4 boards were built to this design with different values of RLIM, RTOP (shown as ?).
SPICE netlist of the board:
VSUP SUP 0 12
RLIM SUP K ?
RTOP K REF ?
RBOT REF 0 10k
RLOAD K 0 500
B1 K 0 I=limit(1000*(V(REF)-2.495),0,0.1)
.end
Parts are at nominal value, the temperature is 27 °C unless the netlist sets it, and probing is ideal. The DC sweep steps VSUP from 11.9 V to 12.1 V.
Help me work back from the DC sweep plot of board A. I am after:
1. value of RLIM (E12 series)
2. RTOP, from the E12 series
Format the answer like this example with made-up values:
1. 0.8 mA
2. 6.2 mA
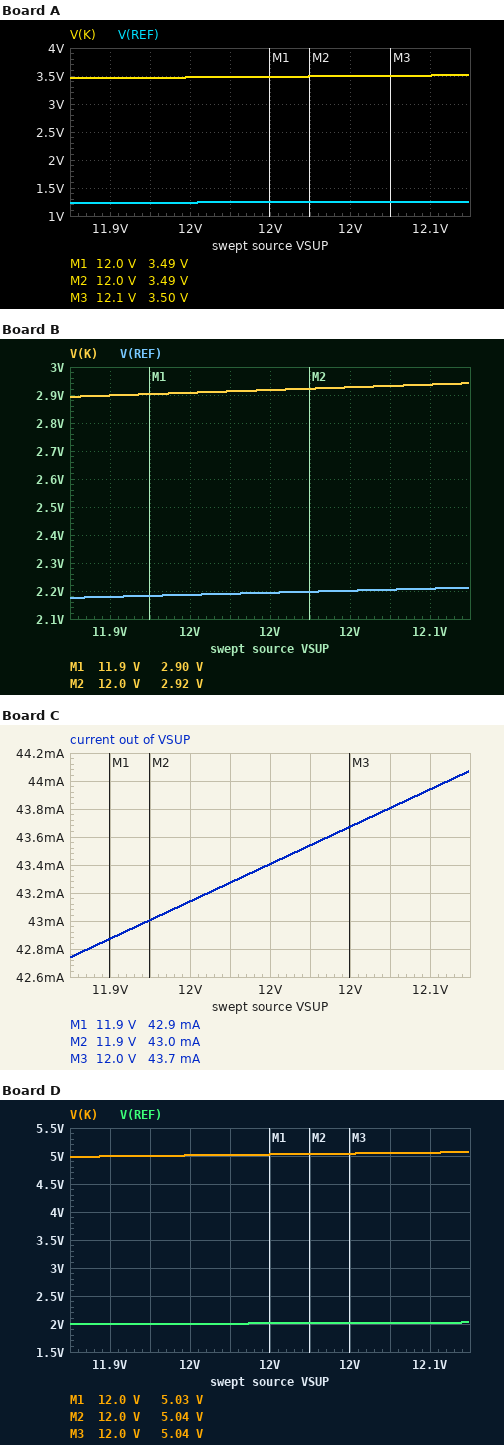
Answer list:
1. 1.2 kΩ
2. 18 kΩ
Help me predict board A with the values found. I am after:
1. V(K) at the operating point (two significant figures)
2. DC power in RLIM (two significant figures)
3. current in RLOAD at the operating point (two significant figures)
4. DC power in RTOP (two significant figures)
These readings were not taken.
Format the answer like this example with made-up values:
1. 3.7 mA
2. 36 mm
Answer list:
1. 3.5 V
2. 60 mW
3. 7.0 mA
4. 280 µW
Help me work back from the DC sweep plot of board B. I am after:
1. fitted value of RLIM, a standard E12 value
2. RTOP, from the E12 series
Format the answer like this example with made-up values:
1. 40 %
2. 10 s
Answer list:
1. 1.5 kΩ
2. 3.3 kΩ
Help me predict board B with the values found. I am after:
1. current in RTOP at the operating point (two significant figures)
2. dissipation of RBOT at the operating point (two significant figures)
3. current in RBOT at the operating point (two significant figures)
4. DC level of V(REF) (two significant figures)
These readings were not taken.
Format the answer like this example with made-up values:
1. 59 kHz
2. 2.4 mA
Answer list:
1. 220 µA
2. 480 µW
3. 220 µA
4. 2.2 V
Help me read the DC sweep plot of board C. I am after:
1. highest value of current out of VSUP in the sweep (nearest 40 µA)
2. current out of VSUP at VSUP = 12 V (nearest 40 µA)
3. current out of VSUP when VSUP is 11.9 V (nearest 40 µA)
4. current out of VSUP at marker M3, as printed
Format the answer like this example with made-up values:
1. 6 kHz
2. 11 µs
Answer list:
1. 44.08 mA
2. 43.68 mA
3. 43.00 mA
4. 43.7 mA
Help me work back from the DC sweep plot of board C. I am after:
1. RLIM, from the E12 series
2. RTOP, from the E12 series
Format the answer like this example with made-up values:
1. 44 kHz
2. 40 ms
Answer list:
1. 150 Ω
2. 12 kΩ
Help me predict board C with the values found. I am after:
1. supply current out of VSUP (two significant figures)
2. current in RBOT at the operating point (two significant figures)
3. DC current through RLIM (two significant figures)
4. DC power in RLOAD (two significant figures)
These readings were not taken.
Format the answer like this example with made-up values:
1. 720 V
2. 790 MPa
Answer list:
1. 43 mA
2. 250 µA
3. 43 mA
4. 60 mW
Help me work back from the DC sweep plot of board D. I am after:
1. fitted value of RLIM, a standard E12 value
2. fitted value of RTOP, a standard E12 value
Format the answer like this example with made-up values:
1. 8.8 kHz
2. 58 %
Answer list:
1. 680 Ω
2. 15 kΩ
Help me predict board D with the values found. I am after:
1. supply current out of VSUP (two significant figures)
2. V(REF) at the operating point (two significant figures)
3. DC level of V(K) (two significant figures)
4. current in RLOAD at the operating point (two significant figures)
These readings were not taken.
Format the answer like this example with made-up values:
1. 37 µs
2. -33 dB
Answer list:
1. 10 mA
2. 2.0 V
3. 5.0 V
4. 10 mA
